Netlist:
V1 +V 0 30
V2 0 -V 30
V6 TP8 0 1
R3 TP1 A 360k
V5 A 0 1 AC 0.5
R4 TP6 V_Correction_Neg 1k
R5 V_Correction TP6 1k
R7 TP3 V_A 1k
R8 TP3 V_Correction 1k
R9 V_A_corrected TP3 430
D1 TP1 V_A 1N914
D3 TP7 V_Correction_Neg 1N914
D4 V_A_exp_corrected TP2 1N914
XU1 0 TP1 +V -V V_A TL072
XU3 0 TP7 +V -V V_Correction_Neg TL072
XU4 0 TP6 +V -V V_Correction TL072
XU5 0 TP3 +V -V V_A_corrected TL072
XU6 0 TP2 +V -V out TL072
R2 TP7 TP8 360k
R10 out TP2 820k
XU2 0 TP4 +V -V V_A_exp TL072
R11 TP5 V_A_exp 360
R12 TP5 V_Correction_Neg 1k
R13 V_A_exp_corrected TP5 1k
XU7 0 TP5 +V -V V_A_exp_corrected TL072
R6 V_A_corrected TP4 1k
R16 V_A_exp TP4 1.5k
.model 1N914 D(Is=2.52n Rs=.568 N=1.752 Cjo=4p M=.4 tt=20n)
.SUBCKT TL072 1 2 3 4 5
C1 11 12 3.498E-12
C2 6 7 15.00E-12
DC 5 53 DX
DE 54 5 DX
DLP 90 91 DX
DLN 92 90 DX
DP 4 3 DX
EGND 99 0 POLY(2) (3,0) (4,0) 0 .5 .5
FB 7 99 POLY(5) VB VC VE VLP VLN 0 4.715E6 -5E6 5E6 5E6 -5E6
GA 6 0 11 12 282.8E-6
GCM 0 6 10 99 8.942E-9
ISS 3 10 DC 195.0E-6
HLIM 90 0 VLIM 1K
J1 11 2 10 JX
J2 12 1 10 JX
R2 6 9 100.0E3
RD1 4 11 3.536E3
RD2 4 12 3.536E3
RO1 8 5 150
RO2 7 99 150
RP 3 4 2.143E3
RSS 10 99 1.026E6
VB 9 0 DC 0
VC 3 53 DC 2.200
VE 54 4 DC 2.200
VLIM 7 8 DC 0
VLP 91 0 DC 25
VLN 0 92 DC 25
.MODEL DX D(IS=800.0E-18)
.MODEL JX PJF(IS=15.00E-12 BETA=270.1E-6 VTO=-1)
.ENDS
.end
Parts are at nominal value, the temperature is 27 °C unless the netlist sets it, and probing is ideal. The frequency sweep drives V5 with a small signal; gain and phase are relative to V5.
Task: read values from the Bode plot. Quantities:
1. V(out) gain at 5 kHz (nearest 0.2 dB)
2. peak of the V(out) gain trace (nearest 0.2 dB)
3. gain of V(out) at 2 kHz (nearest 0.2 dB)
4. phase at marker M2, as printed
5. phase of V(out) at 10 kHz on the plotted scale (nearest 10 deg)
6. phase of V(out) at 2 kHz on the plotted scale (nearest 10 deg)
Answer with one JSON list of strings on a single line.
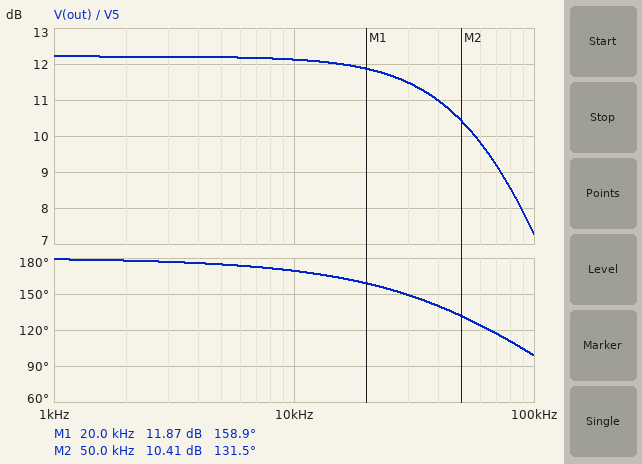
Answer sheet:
["12.2 dB", "12.2 dB", "12.2 dB", "131.5 deg", "170 deg", "180 deg"]
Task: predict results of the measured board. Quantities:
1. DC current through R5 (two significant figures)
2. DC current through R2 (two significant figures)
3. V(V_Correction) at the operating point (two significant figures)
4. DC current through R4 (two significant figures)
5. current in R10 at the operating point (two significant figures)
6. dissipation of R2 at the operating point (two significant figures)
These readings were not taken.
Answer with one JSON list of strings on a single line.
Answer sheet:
["320 µA", "2.8 µA", "320 mV", "320 µA", "2.8 µA", "2.8 µW"]
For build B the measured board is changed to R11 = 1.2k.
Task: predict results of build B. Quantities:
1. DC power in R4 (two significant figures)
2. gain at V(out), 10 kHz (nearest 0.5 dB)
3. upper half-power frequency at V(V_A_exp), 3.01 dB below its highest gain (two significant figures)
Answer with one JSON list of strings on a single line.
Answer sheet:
["100 µW", "1.5 dB", "800 kHz"]
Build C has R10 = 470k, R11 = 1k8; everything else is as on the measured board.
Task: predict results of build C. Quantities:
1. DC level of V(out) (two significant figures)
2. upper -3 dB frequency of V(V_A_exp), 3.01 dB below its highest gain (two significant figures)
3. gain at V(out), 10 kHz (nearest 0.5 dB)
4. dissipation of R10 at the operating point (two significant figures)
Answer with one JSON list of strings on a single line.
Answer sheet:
["-1.3 V", "820 kHz", "-6.5 dB", "3.6 µW"]
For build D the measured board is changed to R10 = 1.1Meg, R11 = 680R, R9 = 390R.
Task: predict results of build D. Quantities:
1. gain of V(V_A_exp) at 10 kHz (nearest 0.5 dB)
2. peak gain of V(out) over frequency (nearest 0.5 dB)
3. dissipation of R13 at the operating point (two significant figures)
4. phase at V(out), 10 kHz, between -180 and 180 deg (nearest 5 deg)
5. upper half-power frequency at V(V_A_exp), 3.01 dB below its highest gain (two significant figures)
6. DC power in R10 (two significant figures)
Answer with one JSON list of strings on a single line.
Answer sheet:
["-31.5 dB", "8.5 dB", "100 µW", "165 deg", "770 kHz", "8.5 µW"]
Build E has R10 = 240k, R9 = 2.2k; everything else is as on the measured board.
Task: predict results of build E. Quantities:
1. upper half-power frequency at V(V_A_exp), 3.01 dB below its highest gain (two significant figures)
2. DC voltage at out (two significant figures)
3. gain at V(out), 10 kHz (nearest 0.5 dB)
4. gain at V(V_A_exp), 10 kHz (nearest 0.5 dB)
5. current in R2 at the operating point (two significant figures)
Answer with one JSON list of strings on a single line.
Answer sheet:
["410 kHz", "-670 mV", "15.5 dB", "-16.5 dB", "2.8 µA"]
